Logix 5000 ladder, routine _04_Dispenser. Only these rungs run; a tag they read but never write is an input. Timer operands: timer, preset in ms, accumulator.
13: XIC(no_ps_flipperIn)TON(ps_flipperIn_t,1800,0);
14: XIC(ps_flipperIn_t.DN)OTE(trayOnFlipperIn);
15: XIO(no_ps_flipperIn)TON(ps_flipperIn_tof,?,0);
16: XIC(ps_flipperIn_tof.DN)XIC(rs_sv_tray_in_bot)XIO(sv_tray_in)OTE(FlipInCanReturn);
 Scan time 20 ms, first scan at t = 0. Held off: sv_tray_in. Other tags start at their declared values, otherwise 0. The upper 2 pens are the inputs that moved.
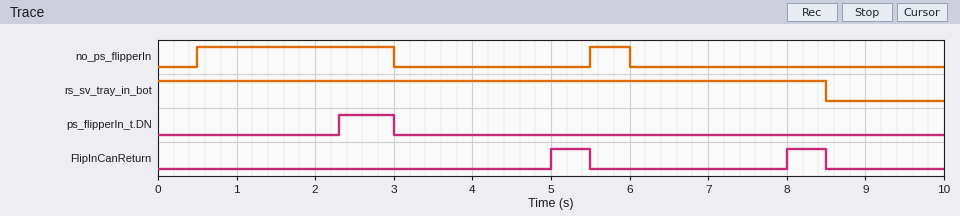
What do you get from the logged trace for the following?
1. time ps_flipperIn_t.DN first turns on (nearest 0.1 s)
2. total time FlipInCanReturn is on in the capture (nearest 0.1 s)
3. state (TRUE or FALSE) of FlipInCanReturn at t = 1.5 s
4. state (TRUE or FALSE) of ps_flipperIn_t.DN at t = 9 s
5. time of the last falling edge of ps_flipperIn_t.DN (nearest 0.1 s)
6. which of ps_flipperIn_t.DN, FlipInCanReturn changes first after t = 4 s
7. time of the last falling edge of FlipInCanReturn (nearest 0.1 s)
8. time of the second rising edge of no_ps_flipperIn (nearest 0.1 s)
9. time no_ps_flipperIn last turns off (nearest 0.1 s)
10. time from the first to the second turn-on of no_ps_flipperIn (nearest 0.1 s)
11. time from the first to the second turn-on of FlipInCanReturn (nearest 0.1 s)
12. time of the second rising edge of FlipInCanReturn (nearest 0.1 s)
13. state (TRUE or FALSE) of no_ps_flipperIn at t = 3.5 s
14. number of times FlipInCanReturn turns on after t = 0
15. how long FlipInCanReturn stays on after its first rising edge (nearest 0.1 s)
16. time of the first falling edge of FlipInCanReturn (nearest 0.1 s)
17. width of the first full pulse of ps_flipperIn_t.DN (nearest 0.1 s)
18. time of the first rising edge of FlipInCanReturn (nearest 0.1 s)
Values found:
2.3 s
1.0 s
FALSE
FALSE
3.0 s
FlipInCanReturn
8.5 s
5.5 s
6.0 s
5.0 s
3.0 s
8.0 s
FALSE
2
0.5 s
5.5 s
0.7 s
5.0 s
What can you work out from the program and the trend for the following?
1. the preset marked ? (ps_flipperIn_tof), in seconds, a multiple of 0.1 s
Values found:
2.0 s
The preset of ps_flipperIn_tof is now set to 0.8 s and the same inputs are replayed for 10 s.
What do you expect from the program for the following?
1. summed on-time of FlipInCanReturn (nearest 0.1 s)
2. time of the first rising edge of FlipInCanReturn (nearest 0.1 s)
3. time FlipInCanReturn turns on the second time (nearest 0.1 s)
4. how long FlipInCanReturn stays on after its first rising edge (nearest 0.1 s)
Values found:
3.4 s
3.8 s
6.8 s
1.7 s
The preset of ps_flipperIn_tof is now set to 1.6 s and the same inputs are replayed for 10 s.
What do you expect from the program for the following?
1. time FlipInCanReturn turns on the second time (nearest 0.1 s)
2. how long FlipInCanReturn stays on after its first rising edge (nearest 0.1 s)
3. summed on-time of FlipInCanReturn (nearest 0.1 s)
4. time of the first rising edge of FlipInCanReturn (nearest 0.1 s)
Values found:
7.6 s
0.9 s
1.8 s
4.6 s
